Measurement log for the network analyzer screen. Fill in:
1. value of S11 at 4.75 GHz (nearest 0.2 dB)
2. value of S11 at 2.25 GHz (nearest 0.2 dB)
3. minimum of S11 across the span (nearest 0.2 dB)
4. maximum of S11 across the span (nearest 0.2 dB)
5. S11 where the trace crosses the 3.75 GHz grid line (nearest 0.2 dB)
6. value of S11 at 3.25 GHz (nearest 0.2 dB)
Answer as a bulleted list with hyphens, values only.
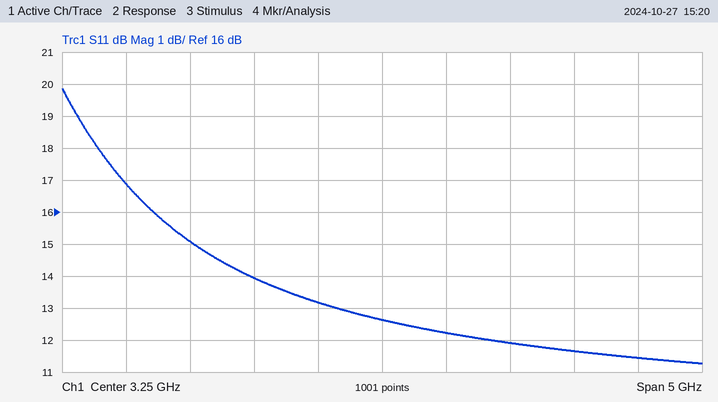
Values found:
- 11.6 dB
- 14.0 dB
- 11.2 dB
- 19.8 dB
- 12.2 dB
- 12.6 dB
